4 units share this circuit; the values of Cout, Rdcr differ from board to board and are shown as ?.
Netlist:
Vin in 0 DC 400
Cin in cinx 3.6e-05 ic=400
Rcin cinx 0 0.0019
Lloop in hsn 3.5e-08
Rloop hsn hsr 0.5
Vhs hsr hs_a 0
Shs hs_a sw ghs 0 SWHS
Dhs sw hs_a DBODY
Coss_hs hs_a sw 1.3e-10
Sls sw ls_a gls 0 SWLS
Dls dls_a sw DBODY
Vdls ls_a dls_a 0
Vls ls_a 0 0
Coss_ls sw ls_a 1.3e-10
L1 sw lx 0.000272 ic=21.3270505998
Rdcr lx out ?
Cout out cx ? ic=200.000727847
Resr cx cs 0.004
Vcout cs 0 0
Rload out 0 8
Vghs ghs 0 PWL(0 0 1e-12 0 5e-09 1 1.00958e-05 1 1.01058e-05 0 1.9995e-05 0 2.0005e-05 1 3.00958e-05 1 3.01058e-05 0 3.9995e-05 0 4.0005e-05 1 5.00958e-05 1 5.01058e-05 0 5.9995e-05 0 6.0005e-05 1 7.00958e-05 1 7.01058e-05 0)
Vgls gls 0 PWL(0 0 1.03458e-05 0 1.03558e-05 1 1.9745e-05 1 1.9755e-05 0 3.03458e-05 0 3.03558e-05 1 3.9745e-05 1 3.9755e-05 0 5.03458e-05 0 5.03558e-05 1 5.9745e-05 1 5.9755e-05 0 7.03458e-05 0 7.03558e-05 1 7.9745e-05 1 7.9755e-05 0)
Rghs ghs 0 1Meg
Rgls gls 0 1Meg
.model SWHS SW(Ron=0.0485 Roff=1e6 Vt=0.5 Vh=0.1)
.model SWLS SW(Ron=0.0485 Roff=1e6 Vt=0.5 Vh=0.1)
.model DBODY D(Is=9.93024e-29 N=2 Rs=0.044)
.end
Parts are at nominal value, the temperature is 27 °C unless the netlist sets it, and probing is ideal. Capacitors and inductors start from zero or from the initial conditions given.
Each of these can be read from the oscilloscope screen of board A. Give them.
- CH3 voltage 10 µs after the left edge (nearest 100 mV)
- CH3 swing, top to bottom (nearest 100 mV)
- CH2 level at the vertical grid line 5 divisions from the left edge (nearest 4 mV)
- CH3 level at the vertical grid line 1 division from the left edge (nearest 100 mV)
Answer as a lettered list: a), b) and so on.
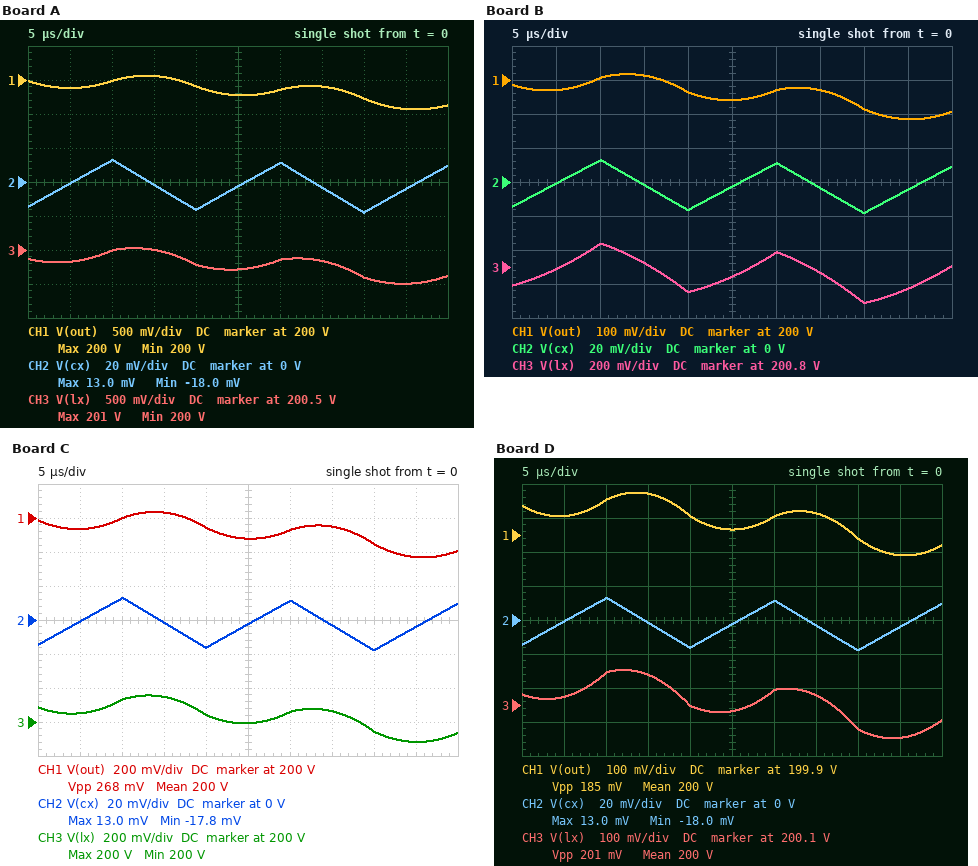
a) 200.5 V
b) 500 mV
c) -4 mV
d) 200.3 V
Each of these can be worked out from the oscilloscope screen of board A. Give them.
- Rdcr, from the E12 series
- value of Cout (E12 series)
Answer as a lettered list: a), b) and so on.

a) 0.018 Ω
b) 82 µF
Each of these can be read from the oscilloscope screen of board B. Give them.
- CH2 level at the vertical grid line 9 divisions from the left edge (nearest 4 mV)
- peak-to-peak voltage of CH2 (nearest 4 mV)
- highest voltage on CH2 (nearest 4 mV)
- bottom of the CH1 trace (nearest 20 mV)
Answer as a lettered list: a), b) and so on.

a) -4 mV
b) 32 mV
c) 12 mV
d) 199.88 V
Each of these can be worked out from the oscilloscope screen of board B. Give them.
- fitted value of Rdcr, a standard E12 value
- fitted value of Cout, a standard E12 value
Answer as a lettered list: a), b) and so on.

a) 0.033 Ω
b) 330 µF
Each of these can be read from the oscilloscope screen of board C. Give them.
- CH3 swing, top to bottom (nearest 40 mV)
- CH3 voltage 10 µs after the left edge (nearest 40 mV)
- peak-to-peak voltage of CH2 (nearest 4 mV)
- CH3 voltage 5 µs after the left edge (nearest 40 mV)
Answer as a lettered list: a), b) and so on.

a) 280 mV
b) 200.12 V
c) 32 mV
d) 200.04 V
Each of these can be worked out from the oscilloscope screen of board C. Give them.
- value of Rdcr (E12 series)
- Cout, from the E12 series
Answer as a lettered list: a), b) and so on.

a) 4.7 mΩ
b) 150 µF
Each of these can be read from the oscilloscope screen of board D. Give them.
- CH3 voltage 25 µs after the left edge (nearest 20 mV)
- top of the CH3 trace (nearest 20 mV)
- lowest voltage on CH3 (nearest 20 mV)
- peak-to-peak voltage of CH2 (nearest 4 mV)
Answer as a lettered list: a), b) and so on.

a) 200.08 V
b) 200.20 V
c) 200.00 V
d) 32 mV
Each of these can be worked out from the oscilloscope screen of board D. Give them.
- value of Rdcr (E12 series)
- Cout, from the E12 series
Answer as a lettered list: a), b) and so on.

a) 6.8 mΩ
b) 220 µF
